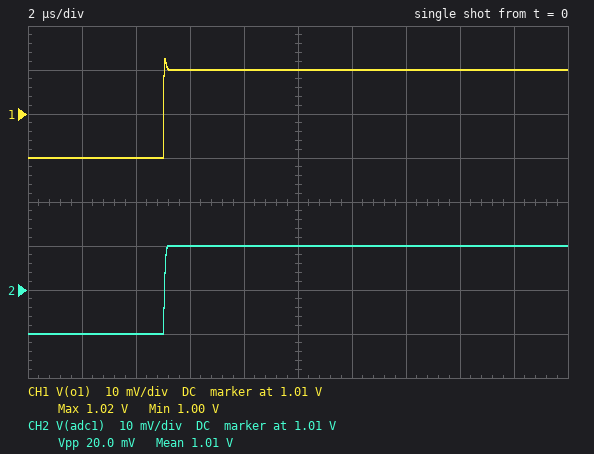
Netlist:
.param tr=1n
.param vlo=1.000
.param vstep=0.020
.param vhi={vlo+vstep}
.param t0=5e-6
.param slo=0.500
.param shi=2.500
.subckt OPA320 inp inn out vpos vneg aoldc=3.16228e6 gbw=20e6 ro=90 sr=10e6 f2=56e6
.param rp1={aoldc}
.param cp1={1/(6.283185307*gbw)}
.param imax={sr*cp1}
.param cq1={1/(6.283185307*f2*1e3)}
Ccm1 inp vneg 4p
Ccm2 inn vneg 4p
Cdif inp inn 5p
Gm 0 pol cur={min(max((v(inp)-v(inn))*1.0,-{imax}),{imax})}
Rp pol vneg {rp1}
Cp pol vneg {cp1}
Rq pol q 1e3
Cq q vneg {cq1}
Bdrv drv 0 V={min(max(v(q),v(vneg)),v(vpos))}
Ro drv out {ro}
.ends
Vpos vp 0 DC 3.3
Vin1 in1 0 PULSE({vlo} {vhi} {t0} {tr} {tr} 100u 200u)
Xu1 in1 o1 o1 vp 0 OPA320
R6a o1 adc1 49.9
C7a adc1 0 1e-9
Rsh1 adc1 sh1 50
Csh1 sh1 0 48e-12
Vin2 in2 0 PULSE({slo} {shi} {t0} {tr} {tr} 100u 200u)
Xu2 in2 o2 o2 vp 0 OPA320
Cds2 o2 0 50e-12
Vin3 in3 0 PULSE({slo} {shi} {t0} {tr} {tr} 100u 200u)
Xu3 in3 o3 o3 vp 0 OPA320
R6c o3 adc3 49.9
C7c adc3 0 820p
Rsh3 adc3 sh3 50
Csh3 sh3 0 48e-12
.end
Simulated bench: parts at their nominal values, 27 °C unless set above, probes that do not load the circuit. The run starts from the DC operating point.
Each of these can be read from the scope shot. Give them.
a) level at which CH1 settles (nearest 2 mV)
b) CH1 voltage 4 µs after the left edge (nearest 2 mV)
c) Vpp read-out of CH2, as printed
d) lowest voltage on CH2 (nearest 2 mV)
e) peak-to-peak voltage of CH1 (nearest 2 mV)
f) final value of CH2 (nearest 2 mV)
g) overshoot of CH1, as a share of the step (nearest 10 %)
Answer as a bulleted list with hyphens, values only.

- 1.020 V
- 1.000 V
- 20.0 mV
- 1.000 V
- 22 mV
- 1.020 V
- 10 %
